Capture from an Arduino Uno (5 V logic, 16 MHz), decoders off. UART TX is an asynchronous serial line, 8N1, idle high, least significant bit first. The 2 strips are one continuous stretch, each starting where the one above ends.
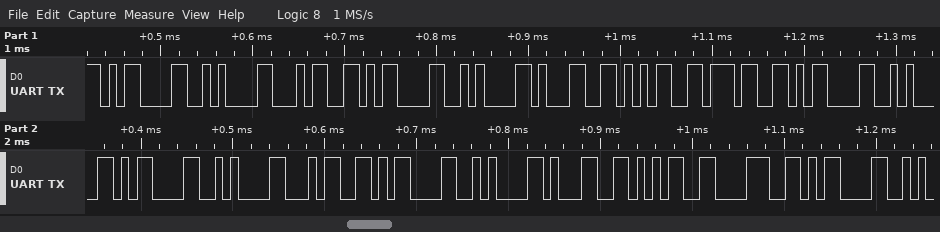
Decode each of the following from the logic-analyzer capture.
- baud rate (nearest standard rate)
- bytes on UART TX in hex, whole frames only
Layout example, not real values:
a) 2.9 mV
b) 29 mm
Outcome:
a) 115200 baud
b) 0D 0A 34 0D 0A 31 35 37 0D 0A 0D 0A 34 0D 0A 31 35 38 0D
